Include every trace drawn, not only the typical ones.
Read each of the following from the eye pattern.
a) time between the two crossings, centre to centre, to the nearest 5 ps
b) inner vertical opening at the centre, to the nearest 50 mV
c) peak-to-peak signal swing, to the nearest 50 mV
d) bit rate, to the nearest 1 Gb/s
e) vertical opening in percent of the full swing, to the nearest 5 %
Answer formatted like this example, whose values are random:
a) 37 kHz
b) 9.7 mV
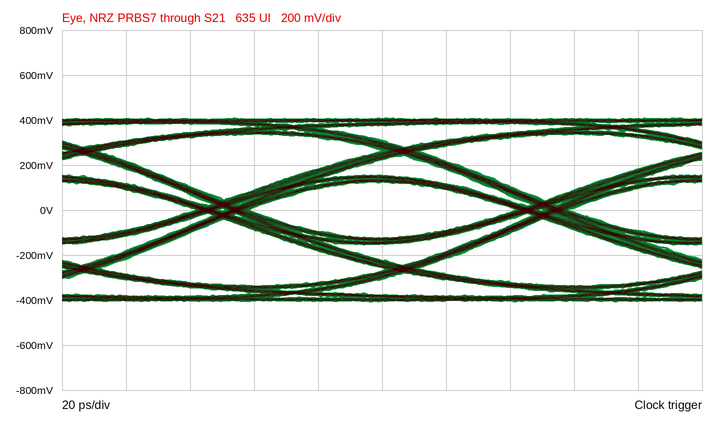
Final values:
a) 100 ps
b) 250 mV
c) 800 mV
d) 10 Gb/s
e) 30 %
